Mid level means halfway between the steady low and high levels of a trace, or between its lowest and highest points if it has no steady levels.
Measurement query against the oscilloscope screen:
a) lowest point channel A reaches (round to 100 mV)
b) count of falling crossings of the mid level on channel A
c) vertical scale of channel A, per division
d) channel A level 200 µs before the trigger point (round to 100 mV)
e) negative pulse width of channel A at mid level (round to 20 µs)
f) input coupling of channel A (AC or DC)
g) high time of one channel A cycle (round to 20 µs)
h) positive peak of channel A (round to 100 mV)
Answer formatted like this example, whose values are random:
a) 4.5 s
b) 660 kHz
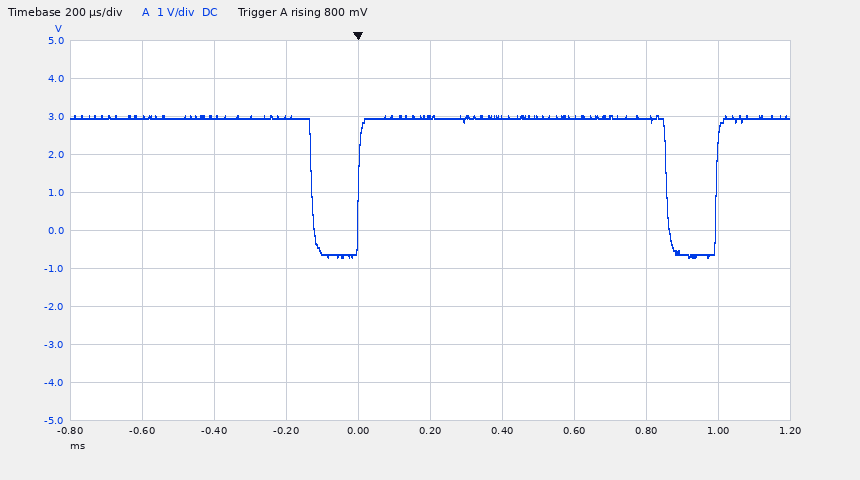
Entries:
a) -700 mV
b) 2
c) 1 V
d) 3.0 V
e) 140 µs
f) DC
g) 860 µs
h) 3.0 V
